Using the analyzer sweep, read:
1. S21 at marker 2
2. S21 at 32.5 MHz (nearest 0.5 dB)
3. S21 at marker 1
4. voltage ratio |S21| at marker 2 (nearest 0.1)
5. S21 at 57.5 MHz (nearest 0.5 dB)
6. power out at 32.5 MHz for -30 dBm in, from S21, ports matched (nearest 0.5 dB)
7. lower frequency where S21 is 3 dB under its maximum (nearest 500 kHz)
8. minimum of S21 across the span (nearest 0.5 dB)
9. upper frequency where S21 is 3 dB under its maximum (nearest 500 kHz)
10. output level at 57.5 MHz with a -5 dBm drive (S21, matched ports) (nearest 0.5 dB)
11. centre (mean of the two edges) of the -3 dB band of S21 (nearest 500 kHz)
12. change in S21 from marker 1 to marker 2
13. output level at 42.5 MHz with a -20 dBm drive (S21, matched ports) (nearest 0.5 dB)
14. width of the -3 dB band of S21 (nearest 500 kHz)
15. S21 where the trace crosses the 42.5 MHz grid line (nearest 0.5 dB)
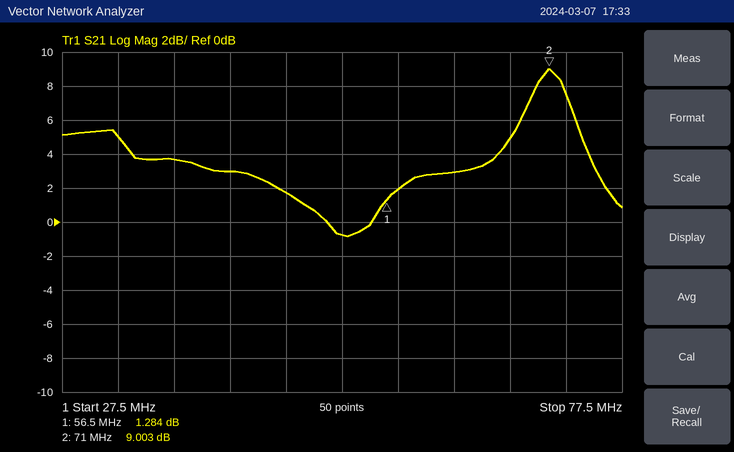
9.003 dB
5.0 dB
1.284 dB
2.8
2.0 dB
-25.0 dBm
68.5 MHz
-1.0 dB
73.5 MHz
-3.0 dBm
71.0 MHz
7.719 dB
-17.0 dBm
5.0 MHz
3.0 dB
